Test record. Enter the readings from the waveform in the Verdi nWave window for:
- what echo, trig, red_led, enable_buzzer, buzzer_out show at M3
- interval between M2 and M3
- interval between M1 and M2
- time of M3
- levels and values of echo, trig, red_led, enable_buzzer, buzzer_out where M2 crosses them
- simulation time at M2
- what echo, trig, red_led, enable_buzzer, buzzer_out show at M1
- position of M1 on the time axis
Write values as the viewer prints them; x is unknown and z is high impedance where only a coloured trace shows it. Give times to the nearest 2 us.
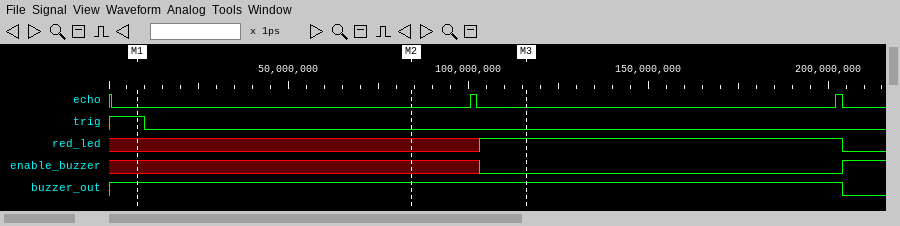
echo=0, trig=0, red_led=1, enable_buzzer=0, buzzer_out=1
32 us
76 us
116 us
echo=0, trig=0, red_led=x, enable_buzzer=x, buzzer_out=1
84 us
echo=0, trig=1, red_led=x, enable_buzzer=x, buzzer_out=1
8 us
